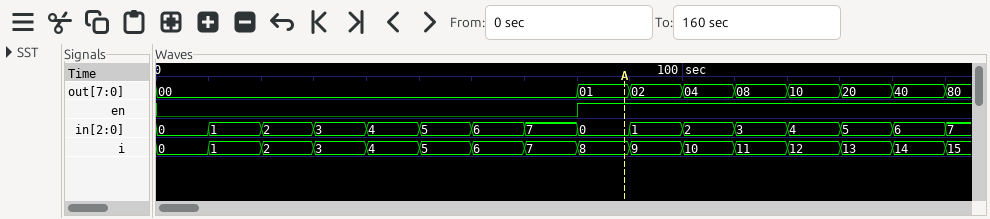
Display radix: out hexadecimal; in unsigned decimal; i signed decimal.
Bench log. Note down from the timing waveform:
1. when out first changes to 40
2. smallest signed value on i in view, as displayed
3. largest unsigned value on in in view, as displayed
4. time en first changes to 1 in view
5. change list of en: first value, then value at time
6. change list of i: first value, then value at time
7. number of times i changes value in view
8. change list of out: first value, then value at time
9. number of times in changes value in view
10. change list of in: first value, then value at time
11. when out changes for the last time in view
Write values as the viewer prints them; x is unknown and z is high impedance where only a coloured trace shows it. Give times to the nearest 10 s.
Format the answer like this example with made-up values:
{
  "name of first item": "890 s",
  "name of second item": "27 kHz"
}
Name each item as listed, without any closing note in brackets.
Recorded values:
{
  "when out first changes to 40": "140 s",
  "smallest signed value on i in view, as displayed": "0",
  "largest unsigned value on in in view, as displayed": "7",
  "time en first changes to 1 in view": "80 s",
  "change list of en: first value, then value at time": "0, 1 at 80 s",
  "change list of i: first value, then value at time": "0, 1 at 10 s, 2 at 20 s, 3 at 30 s, 4 at 40 s, 5 at 50 s, 6 at 60 s, 7 at 70 s, 8 at 80 s, 9 at 90 s, 10 at 100 s, 11 at 110 s, 12 at 120 s, 13 at 130 s, 14 at 140 s, 15 at 150 s",
  "number of times i changes value in view": "15",
  "change list of out: first value, then value at time": "00, 01 at 80 s, 02 at 90 s, 04 at 100 s, 08 at 110 s, 10 at 120 s, 20 at 130 s, 40 at 140 s, 80 at 150 s",
  "number of times in changes value in view": "15",
  "change list of in: first value, then value at time": "0, 1 at 10 s, 2 at 20 s, 3 at 30 s, 4 at 40 s, 5 at 50 s, 6 at 60 s, 7 at 70 s, 0 at 80 s, 1 at 90 s, 2 at 100 s, 3 at 110 s, 4 at 120 s, 5 at 130 s, 6 at 140 s, 7 at 150 s",
  "when out changes for the last time in view": "150 s"
}
